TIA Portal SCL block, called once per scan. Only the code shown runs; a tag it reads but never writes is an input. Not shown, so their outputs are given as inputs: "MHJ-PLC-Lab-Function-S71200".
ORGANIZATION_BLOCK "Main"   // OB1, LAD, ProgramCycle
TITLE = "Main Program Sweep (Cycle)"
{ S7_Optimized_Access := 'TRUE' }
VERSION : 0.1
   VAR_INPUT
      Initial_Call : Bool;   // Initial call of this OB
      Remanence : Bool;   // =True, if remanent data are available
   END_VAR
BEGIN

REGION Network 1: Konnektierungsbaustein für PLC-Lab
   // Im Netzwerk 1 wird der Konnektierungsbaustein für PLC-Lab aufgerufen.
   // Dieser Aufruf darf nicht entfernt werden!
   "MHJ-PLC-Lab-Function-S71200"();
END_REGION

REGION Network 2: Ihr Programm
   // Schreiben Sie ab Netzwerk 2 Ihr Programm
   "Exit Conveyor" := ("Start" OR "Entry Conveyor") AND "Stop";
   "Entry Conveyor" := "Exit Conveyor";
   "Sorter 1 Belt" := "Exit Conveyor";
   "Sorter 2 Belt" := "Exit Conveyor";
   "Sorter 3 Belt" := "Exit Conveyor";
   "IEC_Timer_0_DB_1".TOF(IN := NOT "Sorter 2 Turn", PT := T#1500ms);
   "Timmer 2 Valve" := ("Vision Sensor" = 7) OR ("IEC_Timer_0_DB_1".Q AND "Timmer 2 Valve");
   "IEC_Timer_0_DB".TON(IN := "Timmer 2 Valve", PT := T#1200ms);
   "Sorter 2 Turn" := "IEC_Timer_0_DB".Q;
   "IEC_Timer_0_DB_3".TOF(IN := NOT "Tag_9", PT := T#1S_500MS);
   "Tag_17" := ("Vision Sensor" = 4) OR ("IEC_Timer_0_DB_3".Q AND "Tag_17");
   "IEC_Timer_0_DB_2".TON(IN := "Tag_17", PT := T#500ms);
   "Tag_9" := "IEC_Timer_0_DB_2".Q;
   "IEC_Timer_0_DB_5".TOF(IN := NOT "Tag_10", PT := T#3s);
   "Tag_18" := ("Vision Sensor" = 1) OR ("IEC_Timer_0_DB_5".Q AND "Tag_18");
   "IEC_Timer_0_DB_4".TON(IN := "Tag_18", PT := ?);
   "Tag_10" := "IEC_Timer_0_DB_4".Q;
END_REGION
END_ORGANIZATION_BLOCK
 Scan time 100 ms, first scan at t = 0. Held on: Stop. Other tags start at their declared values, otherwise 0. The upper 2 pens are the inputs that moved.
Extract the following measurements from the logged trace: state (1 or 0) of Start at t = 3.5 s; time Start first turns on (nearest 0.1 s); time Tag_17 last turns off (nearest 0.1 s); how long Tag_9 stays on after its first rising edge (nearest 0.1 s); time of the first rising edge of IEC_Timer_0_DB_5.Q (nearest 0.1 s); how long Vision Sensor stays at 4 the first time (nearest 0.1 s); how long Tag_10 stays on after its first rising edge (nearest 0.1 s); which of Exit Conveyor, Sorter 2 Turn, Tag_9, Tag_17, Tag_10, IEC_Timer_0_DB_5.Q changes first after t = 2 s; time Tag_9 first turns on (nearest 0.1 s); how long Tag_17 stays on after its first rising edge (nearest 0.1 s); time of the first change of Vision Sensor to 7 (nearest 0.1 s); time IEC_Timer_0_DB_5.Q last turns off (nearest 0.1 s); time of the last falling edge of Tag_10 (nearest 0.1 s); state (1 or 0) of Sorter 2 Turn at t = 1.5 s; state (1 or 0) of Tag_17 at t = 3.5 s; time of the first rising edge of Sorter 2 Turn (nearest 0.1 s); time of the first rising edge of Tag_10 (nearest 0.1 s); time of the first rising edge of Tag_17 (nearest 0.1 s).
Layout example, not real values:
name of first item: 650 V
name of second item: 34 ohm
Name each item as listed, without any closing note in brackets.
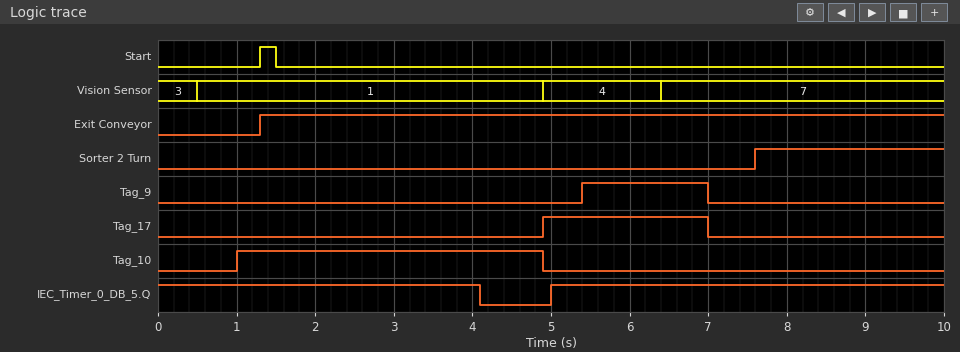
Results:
state (1 or 0) of Start at t = 3.5 s: 0
time Start first turns on: 1.3 s
time Tag_17 last turns off: 7.0 s
how long Tag_9 stays on after its first rising edge: 1.6 s
time of the first rising edge of IEC_Timer_0_DB_5.Q: 5.0 s
how long Vision Sensor stays at 4 the first time: 1.5 s
how long Tag_10 stays on after its first rising edge: 3.9 s
which of Exit Conveyor, Sorter 2 Turn, Tag_9, Tag_17, Tag_10, IEC_Timer_0_DB_5.Q changes first after t = 2 s: IEC_Timer_0_DB_5.Q
time Tag_9 first turns on: 5.4 s
how long Tag_17 stays on after its first rising edge: 2.1 s
time of the first change of Vision Sensor to 7: 6.4 s
time IEC_Timer_0_DB_5.Q last turns off: 4.1 s
time of the last falling edge of Tag_10: 4.9 s
state (1 or 0) of Sorter 2 Turn at t = 1.5 s: 0
state (1 or 0) of Tag_17 at t = 3.5 s: 0
time of the first rising edge of Sorter 2 Turn: 7.6 s
time of the first rising edge of Tag_10: 1.0 s
time of the first rising edge of Tag_17: 4.9 s
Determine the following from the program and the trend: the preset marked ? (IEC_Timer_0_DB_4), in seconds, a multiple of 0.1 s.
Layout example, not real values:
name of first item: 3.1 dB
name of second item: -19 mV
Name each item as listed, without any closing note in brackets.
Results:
the preset marked ? (IEC_Timer_0_DB_4), in seconds, a multiple of 0.1 s: 0.5 s
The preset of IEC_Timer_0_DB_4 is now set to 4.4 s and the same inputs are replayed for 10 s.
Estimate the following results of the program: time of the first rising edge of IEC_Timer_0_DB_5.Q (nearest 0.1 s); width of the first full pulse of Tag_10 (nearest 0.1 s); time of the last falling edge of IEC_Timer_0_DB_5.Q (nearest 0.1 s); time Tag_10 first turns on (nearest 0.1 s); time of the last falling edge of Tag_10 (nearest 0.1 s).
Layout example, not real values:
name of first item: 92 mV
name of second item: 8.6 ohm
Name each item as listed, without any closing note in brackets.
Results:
time of the first rising edge of IEC_Timer_0_DB_5.Q: 8.1 s
width of the first full pulse of Tag_10: 3.1 s
time of the last falling edge of IEC_Timer_0_DB_5.Q: 8.0 s
time Tag_10 first turns on: 4.9 s
time of the last falling edge of Tag_10: 8.0 s
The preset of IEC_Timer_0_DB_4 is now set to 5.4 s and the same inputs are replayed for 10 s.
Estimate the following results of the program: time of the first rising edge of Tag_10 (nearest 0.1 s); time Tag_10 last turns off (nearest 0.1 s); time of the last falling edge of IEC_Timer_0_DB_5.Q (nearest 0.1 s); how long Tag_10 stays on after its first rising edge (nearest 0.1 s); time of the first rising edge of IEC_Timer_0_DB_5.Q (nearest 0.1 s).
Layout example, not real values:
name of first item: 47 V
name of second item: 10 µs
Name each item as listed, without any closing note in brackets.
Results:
time of the first rising edge of Tag_10: 5.9 s
time Tag_10 last turns off: 9.0 s
time of the last falling edge of IEC_Timer_0_DB_5.Q: 9.0 s
how long Tag_10 stays on after its first rising edge: 3.1 s
time of the first rising edge of IEC_Timer_0_DB_5.Q: 9.1 s
